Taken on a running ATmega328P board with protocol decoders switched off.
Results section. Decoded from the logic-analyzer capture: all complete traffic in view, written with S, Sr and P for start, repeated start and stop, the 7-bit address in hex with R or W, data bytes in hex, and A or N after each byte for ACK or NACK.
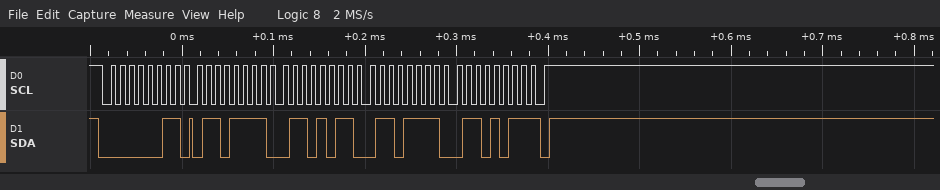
S 01R A 6F A 6B A 6F A 6B N P
